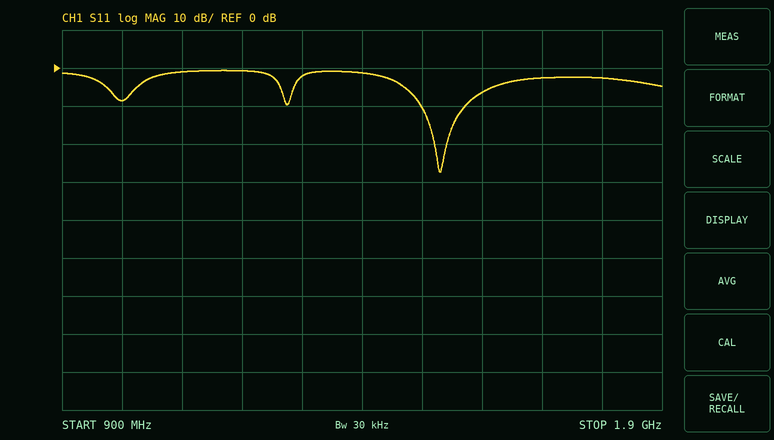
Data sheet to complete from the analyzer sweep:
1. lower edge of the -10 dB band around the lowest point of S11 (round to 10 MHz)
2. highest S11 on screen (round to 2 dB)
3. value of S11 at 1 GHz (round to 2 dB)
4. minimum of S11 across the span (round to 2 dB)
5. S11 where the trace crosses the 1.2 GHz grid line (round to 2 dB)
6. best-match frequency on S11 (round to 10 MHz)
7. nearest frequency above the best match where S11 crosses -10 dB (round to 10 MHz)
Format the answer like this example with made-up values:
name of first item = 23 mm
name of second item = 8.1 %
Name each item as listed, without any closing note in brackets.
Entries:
lower edge of the -10 dB band around the lowest point of S11 = 1.50 GHz
highest S11 on screen = 0 dB
value of S11 at 1 GHz = -8 dB
minimum of S11 across the span = -28 dB
S11 where the trace crosses the 1.2 GHz grid line = 0 dB
best-match frequency on S11 = 1.53 GHz
nearest frequency above the best match where S11 crosses -10 dB = 1.57 GHz
